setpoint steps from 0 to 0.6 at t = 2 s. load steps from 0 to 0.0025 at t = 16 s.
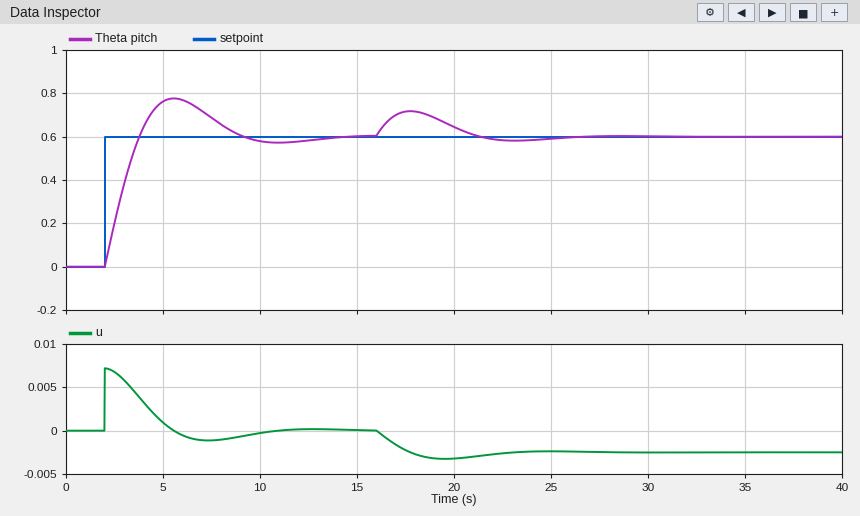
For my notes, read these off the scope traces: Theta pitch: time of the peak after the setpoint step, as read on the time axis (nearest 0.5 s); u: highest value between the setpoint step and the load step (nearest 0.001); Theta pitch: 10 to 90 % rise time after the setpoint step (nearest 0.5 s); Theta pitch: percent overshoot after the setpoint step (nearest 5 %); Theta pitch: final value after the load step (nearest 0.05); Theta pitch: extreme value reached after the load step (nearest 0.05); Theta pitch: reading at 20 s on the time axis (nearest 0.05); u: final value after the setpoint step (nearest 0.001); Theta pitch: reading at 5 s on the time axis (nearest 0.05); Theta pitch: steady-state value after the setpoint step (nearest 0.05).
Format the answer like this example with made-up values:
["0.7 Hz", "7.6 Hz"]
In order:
["5.5 s", "0.007", "1.5 s", "30 %", "0.60", "0.70", "0.65", "0.000", "0.75", "0.60"]
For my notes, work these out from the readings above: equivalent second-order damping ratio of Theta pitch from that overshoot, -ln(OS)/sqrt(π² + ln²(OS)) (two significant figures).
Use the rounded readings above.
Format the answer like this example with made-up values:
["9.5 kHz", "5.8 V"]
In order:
["0.36"]
